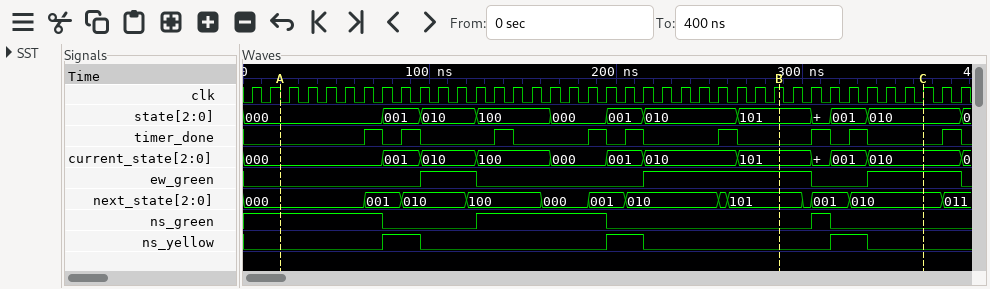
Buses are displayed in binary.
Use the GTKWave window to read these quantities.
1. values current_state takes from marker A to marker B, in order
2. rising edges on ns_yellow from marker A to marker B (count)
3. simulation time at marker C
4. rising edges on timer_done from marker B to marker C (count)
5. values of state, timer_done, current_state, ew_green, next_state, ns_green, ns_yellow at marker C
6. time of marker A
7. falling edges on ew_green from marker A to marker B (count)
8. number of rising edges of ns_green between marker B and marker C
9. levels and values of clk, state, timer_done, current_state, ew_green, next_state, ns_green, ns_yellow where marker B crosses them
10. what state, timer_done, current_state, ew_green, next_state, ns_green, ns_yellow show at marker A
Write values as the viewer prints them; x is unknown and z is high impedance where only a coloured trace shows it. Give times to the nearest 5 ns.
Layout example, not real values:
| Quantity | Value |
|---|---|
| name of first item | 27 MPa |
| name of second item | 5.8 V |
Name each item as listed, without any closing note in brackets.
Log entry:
| Quantity | Value |
|---|---|
| values current_state takes from marker A to marker B, in order | 000, 001, 010, 100, 000, 001, 010, 101 |
| rising edges on ns_yellow from marker A to marker B | 2 |
| simulation time at marker C | 365 ns |
| rising edges on timer_done from marker B to marker C | 2 |
| values of state, timer_done, current_state, ew_green, next_state, ns_green, ns_yellow at marker C | state=010, timer_done=0, current_state=010, ew_green=1, next_state=010, ns_green=0, ns_yellow=0 |
| time of marker A | 20 ns |
| falling edges on ew_green from marker A to marker B | 1 |
| number of rising edges of ns_green between marker B and marker C | 1 |
| levels and values of clk, state, timer_done, current_state, ew_green, next_state, ns_green, ns_yellow where marker B crosses them | clk=1, state=101, timer_done=0, current_state=101, ew_green=1, next_state=101, ns_green=0, ns_yellow=0 |
| what state, timer_done, current_state, ew_green, next_state, ns_green, ns_yellow show at marker A | state=000, timer_done=0, current_state=000, ew_green=0, next_state=000, ns_green=1, ns_yellow=0 |
